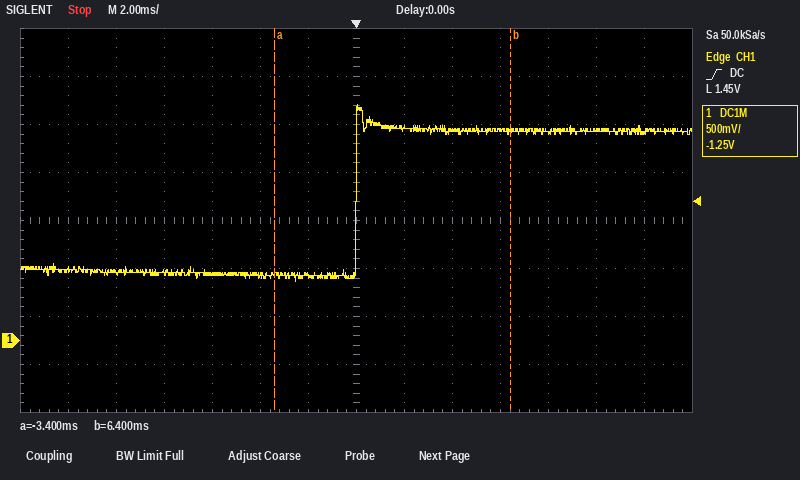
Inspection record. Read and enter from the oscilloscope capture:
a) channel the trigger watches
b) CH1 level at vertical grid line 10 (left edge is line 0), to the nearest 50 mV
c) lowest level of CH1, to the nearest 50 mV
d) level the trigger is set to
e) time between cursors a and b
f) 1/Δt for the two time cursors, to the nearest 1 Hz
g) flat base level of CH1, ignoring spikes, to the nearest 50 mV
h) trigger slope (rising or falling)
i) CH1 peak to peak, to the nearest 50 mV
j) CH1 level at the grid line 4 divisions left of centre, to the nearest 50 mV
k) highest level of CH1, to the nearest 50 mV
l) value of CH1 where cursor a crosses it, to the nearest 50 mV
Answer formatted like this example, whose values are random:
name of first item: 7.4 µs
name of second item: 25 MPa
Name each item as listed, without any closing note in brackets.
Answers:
channel the trigger watches: CH1
CH1 level at vertical grid line 10 (left edge is line 0), to the nearest 50 mV: 2.20 V
lowest level of CH1, to the nearest 50 mV: 600 mV
level the trigger is set to: 1.45 V
time between cursors a and b: 9.8 ms
1/Δt for the two time cursors, to the nearest 1 Hz: 102 Hz
flat base level of CH1, ignoring spikes, to the nearest 50 mV: 700 mV
trigger slope: rising
CH1 peak to peak, to the nearest 50 mV: 1.85 V
CH1 level at the grid line 4 divisions left of centre, to the nearest 50 mV: 700 mV
highest level of CH1, to the nearest 50 mV: 2.45 V
value of CH1 where cursor a crosses it, to the nearest 50 mV: 700 mV
